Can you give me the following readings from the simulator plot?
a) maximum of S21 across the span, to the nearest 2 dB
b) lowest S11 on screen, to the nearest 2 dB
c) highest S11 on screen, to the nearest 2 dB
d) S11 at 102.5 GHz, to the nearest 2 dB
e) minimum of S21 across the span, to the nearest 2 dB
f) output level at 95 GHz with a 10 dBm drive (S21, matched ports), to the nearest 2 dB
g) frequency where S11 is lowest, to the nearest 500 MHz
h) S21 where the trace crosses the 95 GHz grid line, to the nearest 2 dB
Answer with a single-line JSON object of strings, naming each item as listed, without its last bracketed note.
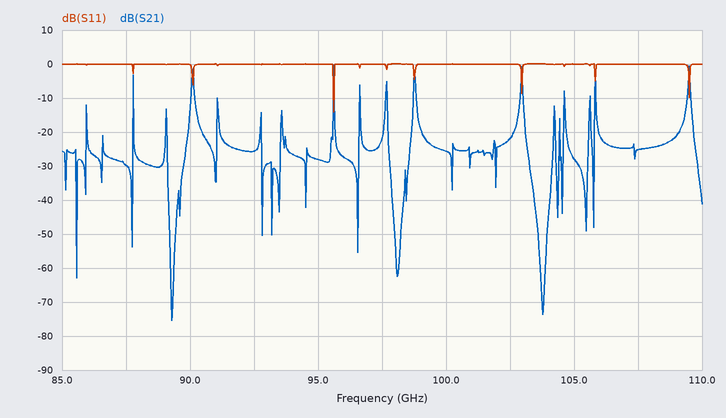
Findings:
{"maximum of S21 across the span, to the nearest 2 dB": "0 dB", "lowest S11 on screen, to the nearest 2 dB": "-14 dB", "highest S11 on screen, to the nearest 2 dB": "0 dB", "S11 at 102.5 GHz, to the nearest 2 dB": "0 dB", "minimum of S21 across the span, to the nearest 2 dB": "-76 dB", "output level at 95 GHz with a 10 dBm drive (S21, matched ports), to the nearest 2 dB": "-18 dBm", "frequency where S11 is lowest, to the nearest 500 MHz": "95.5 GHz", "S21 where the trace crosses the 95 GHz grid line, to the nearest 2 dB": "-28 dB"}
